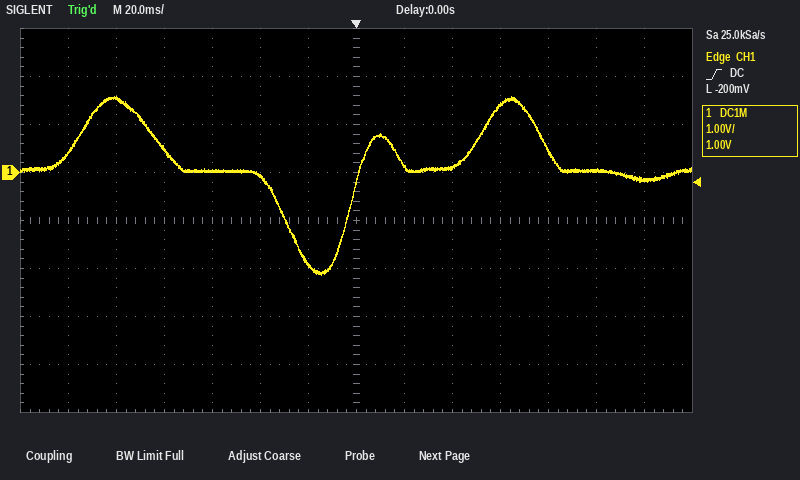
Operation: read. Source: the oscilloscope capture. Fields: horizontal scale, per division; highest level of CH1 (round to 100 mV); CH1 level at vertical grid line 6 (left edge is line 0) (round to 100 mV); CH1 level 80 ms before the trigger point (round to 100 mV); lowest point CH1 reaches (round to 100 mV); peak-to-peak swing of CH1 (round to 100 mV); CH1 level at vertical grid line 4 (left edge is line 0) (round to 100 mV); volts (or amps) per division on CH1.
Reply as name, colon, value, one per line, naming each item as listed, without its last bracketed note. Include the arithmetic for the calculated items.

horizontal scale, per division: 20 ms
highest level of CH1: 1.6 V
CH1 level at vertical grid line 6 (left edge is line 0): -1.9 V
CH1 level 80 ms before the trigger point: 500 mV
lowest point CH1 reaches: -2.1 V
peak-to-peak swing of CH1: 1.6 V − (-2.1 V) = 3.7 V
CH1 level at vertical grid line 4 (left edge is line 0): 0.0 V
volts (or amps) per division on CH1: 1 V
